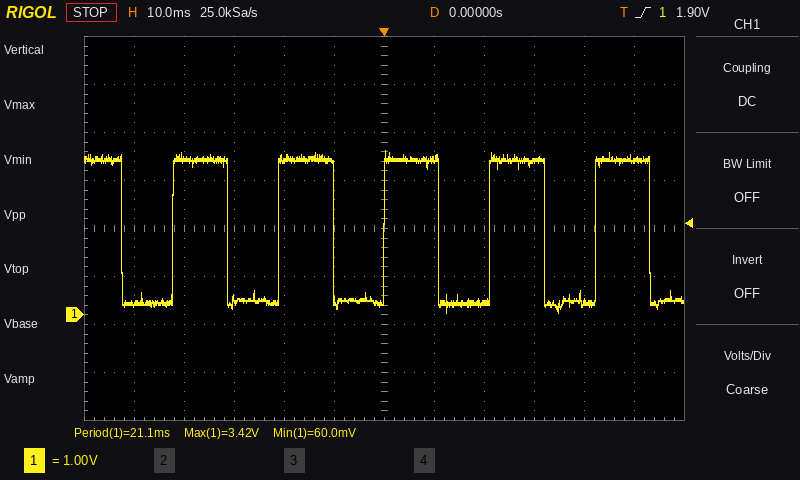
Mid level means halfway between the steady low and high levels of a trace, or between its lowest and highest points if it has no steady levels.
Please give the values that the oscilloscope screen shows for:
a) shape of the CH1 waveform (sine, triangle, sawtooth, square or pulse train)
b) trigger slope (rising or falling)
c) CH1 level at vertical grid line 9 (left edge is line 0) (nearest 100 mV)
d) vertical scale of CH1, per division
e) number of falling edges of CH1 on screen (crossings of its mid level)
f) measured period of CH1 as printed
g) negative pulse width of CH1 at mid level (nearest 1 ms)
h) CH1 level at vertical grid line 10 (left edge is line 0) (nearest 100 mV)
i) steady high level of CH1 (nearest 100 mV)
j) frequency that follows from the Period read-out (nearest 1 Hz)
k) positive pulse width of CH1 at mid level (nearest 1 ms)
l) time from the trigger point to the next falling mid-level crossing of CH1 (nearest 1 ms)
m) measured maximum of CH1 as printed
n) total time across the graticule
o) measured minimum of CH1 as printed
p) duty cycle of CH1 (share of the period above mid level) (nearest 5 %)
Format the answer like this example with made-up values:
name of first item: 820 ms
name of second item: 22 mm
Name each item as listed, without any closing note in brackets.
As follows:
shape of the CH1 waveform: square
trigger slope: rising
CH1 level at vertical grid line 9 (left edge is line 0): 3.2 V
vertical scale of CH1, per division: 1 V
number of falling edges of CH1 on screen: 6
measured period of CH1 as printed: 21.1 ms
negative pulse width of CH1 at mid level: 10 ms
CH1 level at vertical grid line 10 (left edge is line 0): 300 mV
steady high level of CH1: 3.2 V
frequency that follows from the Period read-out: 47 Hz
positive pulse width of CH1 at mid level: 11 ms
time from the trigger point to the next falling mid-level crossing of CH1: 11 ms
measured maximum of CH1 as printed: 3.42 V
total time across the graticule: 120 ms
measured minimum of CH1 as printed: 60.0 mV
duty cycle of CH1 (share of the period above mid level): 50 %
